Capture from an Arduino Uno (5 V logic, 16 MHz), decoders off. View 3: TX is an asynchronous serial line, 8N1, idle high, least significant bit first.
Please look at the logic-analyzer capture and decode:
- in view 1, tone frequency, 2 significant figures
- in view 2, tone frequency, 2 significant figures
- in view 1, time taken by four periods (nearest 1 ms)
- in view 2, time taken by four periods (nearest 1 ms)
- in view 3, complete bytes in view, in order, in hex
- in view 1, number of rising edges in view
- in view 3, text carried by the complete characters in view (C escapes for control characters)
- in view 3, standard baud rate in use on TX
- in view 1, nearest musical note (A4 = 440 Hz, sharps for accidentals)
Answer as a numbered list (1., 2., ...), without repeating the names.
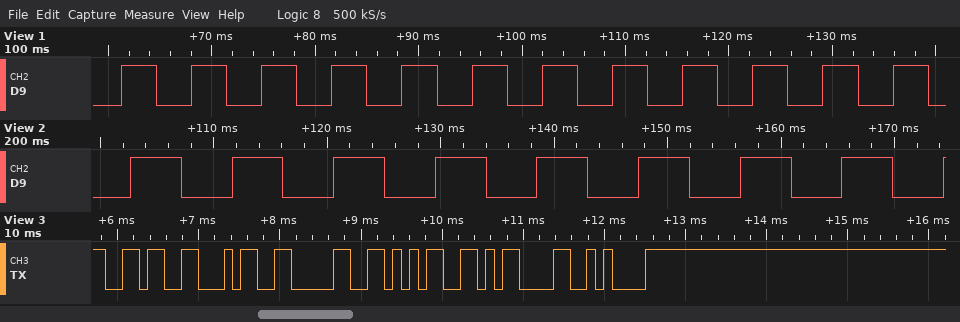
1. 150 Hz
2. 110 Hz
3. 27 ms
4. 36 ms
5. 36 34 30 35 0D 0A
6. 12
7. "6405\r\n"
8. 9600 baud
9. D3
